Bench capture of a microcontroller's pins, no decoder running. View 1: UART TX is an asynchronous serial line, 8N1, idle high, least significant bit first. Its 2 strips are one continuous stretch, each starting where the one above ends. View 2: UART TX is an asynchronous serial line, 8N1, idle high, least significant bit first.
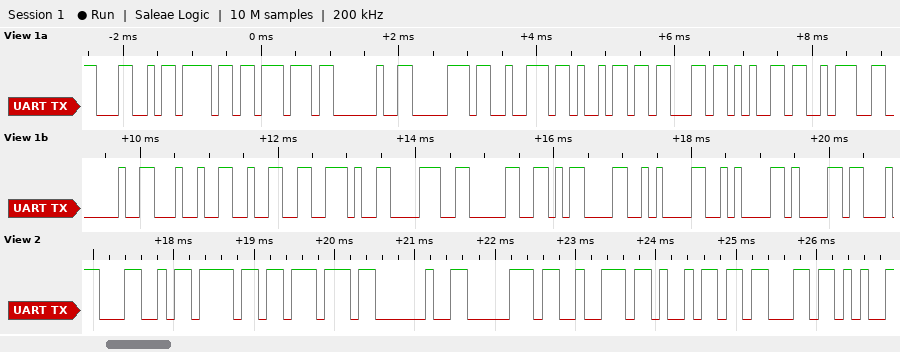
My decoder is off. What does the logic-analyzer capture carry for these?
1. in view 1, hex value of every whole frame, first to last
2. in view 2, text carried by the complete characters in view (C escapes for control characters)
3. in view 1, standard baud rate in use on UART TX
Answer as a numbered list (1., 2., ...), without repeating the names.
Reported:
1. 0x4C 0x6F 0x77 0x20 0x70 0x72 0x69 0x63 0x65 0x3A 0x20 0x24 0x32 0x2E 0x38 0x30 0x0D 0x0A 0x0A 0x61
2. "Low pric"
3. 9600 baud
